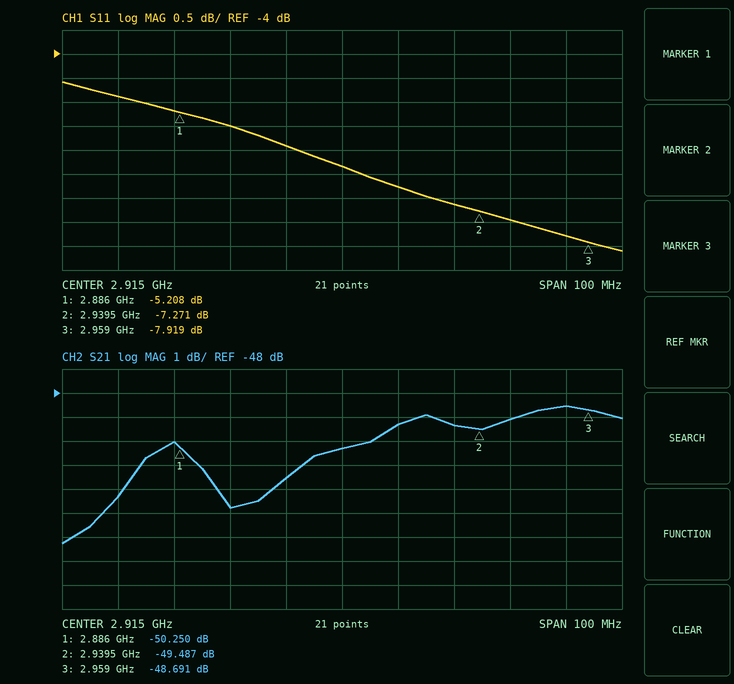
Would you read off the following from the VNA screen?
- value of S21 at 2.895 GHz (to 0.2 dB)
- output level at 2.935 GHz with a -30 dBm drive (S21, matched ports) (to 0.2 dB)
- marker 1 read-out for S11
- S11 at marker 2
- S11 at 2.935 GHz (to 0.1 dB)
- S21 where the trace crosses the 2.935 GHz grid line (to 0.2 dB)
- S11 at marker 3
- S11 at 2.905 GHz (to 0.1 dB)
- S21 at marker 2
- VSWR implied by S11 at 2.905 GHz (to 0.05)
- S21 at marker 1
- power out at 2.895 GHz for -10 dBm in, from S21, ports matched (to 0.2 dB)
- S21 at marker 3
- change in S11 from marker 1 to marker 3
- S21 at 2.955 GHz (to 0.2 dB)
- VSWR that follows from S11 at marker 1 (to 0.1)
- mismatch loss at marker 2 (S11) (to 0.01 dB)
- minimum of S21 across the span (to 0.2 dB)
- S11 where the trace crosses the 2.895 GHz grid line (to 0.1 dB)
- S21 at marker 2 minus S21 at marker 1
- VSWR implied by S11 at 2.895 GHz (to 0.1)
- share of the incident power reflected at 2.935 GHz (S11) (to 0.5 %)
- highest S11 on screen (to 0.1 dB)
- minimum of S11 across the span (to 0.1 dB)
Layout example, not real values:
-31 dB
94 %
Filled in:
-52.8 dB
-79.4 dBm
-5.208 dB
-7.271 dB
-7.1 dB
-49.4 dB
-7.919 dB
-5.9 dB
-49.487 dB
3.05
-50.250 dB
-62.8 dBm
-48.691 dB
-2.711 dB
-48.6 dB
3.4
0.90 dB
-54.2 dB
-5.5 dB
0.763 dB
3.3
19.5 %
-4.6 dB
-8.1 dB
